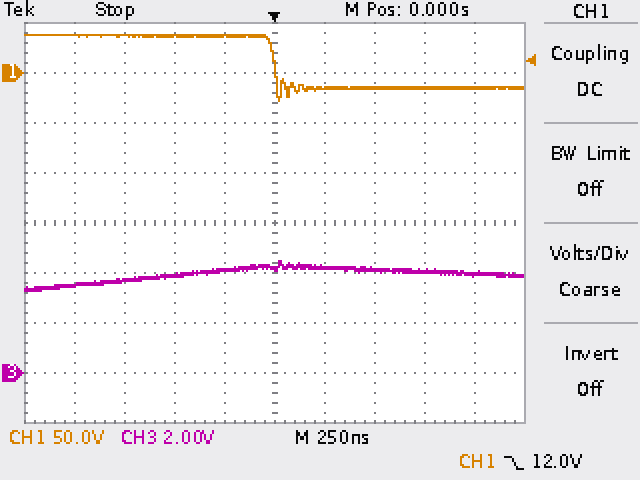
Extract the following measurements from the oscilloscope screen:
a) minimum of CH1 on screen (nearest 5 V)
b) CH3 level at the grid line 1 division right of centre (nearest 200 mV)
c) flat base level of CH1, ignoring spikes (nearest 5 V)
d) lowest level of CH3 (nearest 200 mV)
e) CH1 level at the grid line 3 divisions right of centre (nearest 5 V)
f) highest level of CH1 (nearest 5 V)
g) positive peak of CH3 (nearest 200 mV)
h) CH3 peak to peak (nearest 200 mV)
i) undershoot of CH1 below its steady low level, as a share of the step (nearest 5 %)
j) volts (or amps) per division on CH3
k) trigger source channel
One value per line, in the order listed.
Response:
-30 V
4.2 V
-15 V
3.2 V
-15 V
40 V
4.4 V
1.2 V
25 %
2 V
CH1
